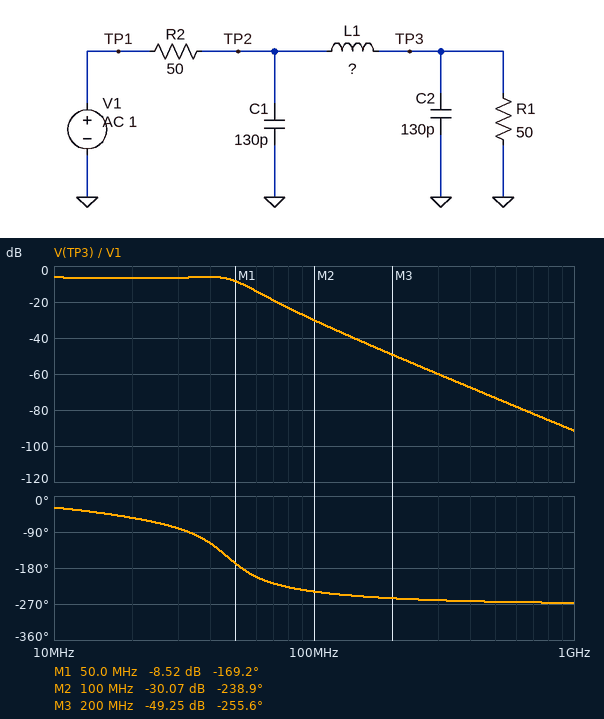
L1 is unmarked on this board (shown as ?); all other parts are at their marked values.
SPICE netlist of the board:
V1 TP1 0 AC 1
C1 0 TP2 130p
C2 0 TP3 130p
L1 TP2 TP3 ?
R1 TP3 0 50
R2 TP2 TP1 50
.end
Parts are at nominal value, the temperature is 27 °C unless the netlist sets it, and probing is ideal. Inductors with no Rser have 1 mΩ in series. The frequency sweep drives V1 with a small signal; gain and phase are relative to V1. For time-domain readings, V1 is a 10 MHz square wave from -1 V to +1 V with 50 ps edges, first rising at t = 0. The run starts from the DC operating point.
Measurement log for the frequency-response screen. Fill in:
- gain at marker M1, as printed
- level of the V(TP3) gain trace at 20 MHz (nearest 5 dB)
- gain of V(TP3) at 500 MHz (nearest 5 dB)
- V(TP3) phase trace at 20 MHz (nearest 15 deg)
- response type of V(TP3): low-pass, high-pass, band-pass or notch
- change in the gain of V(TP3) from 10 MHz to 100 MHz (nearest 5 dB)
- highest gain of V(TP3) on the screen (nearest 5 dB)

-8.52 dB
-5 dB
-75 dB
-60 deg
low-pass
-25 dB
-5 dB
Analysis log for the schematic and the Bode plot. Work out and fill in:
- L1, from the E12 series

180 nH
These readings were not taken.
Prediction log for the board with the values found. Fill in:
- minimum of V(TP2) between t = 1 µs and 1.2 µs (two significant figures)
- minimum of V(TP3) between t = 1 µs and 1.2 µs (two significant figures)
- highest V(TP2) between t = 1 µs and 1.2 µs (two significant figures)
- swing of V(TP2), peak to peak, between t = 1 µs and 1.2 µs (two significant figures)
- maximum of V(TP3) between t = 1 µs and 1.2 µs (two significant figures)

-550 mV
-570 mV
550 mV
1.1 V
570 mV
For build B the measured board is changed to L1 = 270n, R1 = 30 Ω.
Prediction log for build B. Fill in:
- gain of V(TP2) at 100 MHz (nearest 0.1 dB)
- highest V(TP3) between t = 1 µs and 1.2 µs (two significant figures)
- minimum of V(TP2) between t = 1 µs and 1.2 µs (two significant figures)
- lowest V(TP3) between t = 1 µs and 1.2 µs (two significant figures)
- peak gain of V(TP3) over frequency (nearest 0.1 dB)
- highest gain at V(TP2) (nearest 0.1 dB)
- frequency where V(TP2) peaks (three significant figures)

-11.8 dB
460 mV
-690 mV
-460 mV
-8.3 dB
-3.2 dB
36.9 MHz
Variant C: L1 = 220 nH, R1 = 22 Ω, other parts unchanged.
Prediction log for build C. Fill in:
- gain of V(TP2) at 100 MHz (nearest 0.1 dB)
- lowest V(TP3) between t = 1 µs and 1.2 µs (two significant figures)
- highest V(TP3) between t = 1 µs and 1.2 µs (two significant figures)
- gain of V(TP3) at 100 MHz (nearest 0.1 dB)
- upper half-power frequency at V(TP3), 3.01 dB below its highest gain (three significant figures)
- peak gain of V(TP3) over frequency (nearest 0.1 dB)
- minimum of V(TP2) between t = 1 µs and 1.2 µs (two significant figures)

-11.7 dB
-390 mV
390 mV
-33.3 dB
42.6 MHz
-9.7 dB
-700 mV
